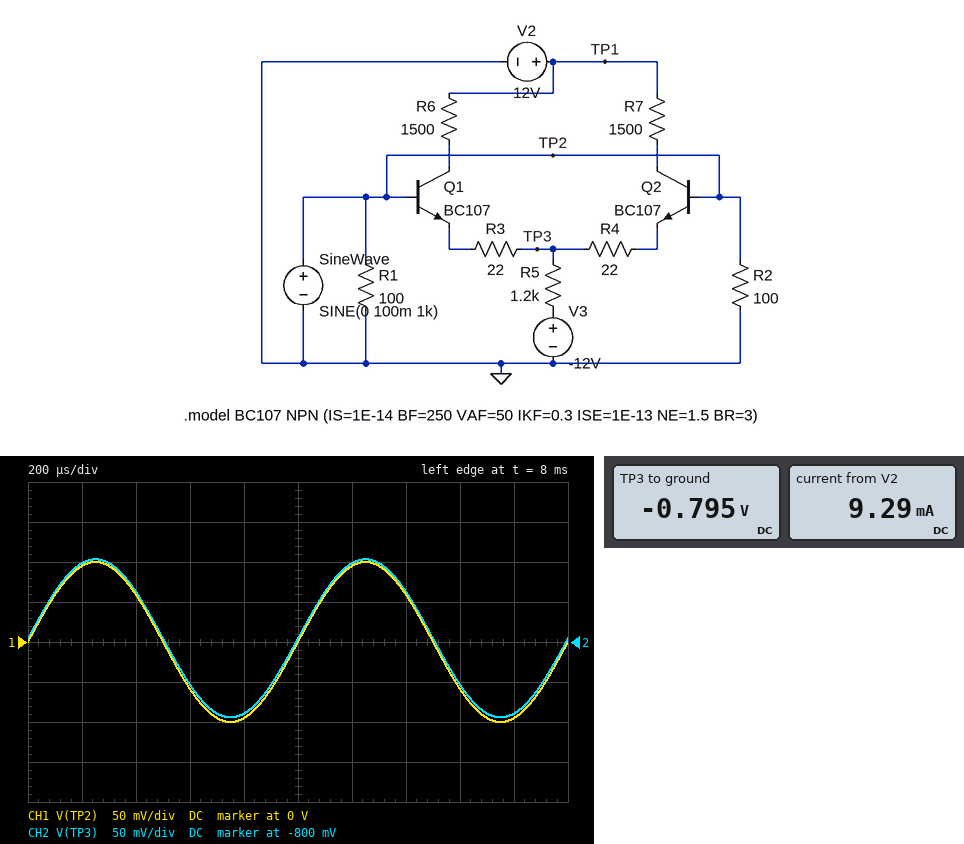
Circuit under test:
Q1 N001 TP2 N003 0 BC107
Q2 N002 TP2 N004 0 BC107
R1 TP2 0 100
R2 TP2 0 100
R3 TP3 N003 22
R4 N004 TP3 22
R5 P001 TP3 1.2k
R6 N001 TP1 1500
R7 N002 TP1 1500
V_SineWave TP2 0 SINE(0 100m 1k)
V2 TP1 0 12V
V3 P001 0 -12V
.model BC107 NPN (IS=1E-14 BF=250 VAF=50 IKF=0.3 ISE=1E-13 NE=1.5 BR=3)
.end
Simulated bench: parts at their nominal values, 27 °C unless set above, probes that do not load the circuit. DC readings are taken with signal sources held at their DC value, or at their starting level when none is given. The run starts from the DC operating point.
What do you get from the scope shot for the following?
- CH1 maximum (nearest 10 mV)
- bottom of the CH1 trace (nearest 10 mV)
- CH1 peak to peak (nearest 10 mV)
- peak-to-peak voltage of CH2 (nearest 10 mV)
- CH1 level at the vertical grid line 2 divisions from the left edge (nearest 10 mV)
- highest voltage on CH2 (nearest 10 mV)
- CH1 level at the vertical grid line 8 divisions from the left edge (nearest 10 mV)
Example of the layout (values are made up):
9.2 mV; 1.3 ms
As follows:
100 mV; -100 mV; 200 mV; 200 mV; 60 mV; -700 mV; -60 mV
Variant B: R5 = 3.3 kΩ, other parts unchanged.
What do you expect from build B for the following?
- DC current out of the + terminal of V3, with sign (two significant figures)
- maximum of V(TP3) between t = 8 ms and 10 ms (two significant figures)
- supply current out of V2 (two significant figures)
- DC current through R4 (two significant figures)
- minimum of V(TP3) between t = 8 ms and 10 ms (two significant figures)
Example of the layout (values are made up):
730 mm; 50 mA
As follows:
-3.4 mA; -600 mV; 3.4 mA; 1.7 mA; -800 mV
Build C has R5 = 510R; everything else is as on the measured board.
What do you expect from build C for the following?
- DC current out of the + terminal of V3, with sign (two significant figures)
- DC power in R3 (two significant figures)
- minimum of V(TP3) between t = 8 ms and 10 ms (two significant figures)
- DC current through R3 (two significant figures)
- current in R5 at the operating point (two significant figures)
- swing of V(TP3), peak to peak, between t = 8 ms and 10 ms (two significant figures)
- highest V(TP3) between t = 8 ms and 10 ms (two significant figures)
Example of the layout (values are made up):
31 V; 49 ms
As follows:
-22 mA; 2.6 mW; -1.1 V; 11 mA; 22 mA; 190 mV; -870 mV
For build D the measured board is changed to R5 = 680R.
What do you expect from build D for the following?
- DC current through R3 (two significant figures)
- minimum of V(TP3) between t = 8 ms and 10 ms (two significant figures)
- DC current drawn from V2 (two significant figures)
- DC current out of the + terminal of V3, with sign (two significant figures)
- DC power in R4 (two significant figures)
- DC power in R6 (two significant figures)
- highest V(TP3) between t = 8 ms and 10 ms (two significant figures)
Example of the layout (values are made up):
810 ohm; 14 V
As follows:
8.2 mA; -990 mV; 16 mA; -16 mA; 1.5 mW; 99 mW; -790 mV
